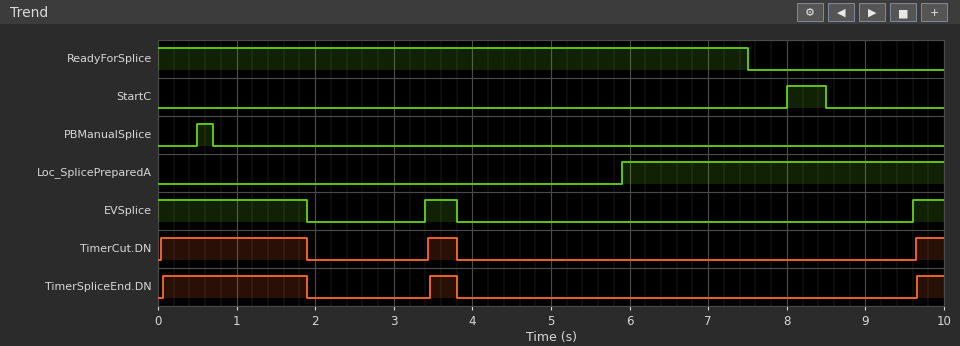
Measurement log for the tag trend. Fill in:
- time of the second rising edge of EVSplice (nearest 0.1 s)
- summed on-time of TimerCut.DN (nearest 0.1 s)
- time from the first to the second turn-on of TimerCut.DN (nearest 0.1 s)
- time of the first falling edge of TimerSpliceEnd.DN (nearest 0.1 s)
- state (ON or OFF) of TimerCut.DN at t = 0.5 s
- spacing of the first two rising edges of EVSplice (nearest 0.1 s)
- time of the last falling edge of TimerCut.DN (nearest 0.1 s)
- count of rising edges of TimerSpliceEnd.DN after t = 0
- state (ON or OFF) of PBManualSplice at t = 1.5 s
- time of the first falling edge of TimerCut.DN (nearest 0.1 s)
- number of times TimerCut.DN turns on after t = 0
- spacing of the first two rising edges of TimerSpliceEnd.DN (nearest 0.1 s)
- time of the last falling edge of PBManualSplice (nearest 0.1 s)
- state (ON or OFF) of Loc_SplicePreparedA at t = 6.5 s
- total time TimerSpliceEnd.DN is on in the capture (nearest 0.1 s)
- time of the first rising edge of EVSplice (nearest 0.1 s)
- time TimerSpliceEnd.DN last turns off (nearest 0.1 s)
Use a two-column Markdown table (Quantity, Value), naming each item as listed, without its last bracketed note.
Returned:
| Quantity | Value |
|---|---|
| time of the second rising edge of EVSplice | 9.6 s |
| summed on-time of TimerCut.DN | 2.6 s |
| time from the first to the second turn-on of TimerCut.DN | 3.4 s |
| time of the first falling edge of TimerSpliceEnd.DN | 1.9 s |
| state (ON or OFF) of TimerCut.DN at t = 0.5 s | ON |
| spacing of the first two rising edges of EVSplice | 6.2 s |
| time of the last falling edge of TimerCut.DN | 3.8 s |
| count of rising edges of TimerSpliceEnd.DN after t = 0 | 3 |
| state (ON or OFF) of PBManualSplice at t = 1.5 s | OFF |
| time of the first falling edge of TimerCut.DN | 1.9 s |
| number of times TimerCut.DN turns on after t = 0 | 3 |
| spacing of the first two rising edges of TimerSpliceEnd.DN | 3.4 s |
| time of the last falling edge of PBManualSplice | 0.7 s |
| state (ON or OFF) of Loc_SplicePreparedA at t = 6.5 s | ON |
| total time TimerSpliceEnd.DN is on in the capture | 2.5 s |
| time of the first rising edge of EVSplice | 3.4 s |
| time TimerSpliceEnd.DN last turns off | 3.8 s |
